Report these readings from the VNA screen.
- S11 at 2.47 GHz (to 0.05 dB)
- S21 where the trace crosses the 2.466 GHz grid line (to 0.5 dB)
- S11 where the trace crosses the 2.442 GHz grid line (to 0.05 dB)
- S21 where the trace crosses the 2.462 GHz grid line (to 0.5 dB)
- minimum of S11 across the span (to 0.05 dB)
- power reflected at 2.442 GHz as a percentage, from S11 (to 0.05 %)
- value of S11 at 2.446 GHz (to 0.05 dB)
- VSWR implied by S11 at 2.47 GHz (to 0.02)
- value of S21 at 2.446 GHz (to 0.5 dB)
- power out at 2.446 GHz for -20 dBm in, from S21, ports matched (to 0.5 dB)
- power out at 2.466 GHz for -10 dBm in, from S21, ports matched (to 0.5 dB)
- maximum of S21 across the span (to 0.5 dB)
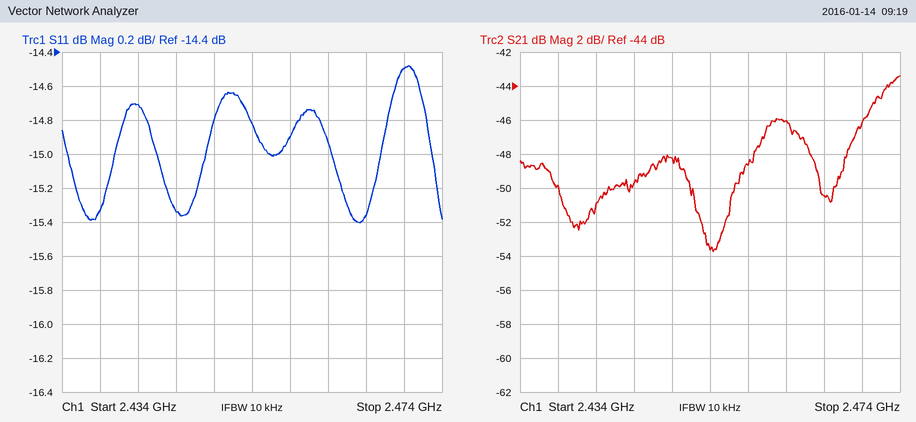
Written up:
-14.50 dB
-50.5 dB
-14.70 dB
-46.0 dB
-15.40 dB
3.40 %
-15.35 dB
1.46
-49.5 dB
-69.5 dBm
-60.5 dBm
-43.5 dB
